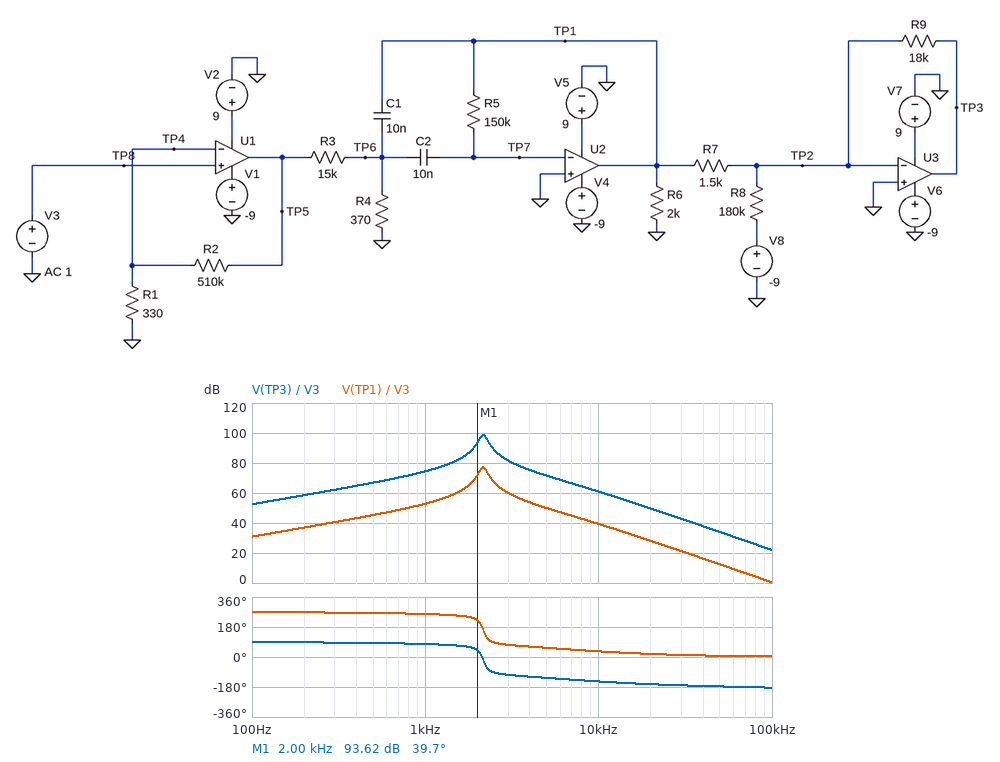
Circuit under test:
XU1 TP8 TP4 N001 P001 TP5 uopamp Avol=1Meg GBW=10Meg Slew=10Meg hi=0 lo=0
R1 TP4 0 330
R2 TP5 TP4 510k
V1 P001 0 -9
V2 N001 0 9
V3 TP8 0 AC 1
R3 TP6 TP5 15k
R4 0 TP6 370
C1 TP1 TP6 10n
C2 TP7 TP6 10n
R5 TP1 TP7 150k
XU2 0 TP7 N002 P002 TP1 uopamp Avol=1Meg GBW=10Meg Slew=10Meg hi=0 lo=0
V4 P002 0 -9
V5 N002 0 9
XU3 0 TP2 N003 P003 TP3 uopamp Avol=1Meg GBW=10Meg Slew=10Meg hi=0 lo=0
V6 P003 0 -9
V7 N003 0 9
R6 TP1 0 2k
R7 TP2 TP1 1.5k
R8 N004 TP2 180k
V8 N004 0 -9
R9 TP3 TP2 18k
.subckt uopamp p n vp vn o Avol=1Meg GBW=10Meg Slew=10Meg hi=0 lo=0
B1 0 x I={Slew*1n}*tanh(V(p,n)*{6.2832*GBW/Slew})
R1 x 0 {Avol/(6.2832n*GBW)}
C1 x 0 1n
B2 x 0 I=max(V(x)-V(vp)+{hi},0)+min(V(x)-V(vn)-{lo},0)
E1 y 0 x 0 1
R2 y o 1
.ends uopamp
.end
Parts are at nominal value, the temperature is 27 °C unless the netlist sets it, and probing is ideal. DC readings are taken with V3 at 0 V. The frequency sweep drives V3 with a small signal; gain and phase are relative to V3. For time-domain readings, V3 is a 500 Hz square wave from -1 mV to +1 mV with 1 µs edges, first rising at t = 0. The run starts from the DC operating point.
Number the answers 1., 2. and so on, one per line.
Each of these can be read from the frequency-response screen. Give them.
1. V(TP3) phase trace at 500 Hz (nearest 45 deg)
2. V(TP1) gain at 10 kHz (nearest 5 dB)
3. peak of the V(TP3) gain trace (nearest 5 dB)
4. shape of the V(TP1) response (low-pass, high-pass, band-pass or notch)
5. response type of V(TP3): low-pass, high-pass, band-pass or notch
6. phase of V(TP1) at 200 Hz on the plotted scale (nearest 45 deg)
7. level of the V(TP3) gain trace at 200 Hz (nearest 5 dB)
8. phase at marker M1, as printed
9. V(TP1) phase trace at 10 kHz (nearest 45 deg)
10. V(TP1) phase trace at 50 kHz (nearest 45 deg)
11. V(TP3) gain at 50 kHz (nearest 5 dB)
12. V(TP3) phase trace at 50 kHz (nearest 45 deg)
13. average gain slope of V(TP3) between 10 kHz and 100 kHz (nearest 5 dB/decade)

1. 90 deg
2. 40 dB
3. 100 dB
4. band-pass
5. band-pass
6. 270 deg
7. 60 dB
8. 39.7 deg
9. 45 deg
10. 0 deg
11. 35 dB
12. -180 deg
13. -40 dB/decade
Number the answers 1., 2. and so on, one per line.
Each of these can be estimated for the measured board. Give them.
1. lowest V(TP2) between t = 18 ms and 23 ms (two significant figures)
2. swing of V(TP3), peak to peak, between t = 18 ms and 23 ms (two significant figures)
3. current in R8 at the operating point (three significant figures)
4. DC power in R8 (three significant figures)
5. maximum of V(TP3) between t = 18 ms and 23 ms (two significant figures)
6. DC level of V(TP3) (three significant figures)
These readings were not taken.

1. -260 mV
2. 18 V
3. 50.0 µA
4. 450 µW
5. 9.0 V
6. 900 mV
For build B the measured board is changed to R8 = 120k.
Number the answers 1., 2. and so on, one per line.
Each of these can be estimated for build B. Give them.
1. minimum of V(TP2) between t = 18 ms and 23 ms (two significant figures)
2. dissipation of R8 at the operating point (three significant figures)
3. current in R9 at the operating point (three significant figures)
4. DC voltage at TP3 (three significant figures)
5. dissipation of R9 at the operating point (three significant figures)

1. -300 mV
2. 675 µW
3. 75.0 µA
4. 1.35 V
5. 101 µW
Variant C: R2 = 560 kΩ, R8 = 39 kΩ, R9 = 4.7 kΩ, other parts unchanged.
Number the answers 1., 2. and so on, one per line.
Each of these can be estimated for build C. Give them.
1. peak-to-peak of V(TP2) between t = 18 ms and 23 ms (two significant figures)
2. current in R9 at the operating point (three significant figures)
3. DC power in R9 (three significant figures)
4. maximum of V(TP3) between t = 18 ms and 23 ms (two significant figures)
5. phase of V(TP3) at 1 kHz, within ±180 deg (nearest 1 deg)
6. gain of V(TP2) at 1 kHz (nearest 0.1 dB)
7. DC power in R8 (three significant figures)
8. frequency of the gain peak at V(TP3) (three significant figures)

1. 1.3 mV
2. 231 µA
3. 250 µW
4. 4.4 V
5. 77 deg
6. -16.4 dB
7. 2.08 mW
8. 2.16 kHz
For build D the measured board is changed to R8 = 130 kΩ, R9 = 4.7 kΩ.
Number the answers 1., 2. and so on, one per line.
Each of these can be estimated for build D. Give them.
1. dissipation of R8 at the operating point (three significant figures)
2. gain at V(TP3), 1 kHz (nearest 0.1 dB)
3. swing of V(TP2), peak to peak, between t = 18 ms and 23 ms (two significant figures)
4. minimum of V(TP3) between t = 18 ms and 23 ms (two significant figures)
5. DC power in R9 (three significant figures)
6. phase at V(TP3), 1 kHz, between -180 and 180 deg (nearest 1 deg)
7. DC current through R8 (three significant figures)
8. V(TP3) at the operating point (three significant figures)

1. 623 µW
2. 62.8 dB
3. 1.2 mV
4. -2.7 V
5. 22.5 µW
6. 78 deg
7. 69.2 µA
8. 325 mV
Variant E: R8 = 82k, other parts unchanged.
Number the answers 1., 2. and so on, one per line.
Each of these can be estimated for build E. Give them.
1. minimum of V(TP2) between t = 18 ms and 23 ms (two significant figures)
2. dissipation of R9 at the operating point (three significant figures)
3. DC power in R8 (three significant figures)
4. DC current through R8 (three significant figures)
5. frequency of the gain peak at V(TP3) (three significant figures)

1. -340 mV
2. 217 µW
3. 988 µW
4. 110 µA
5. 2.16 kHz
